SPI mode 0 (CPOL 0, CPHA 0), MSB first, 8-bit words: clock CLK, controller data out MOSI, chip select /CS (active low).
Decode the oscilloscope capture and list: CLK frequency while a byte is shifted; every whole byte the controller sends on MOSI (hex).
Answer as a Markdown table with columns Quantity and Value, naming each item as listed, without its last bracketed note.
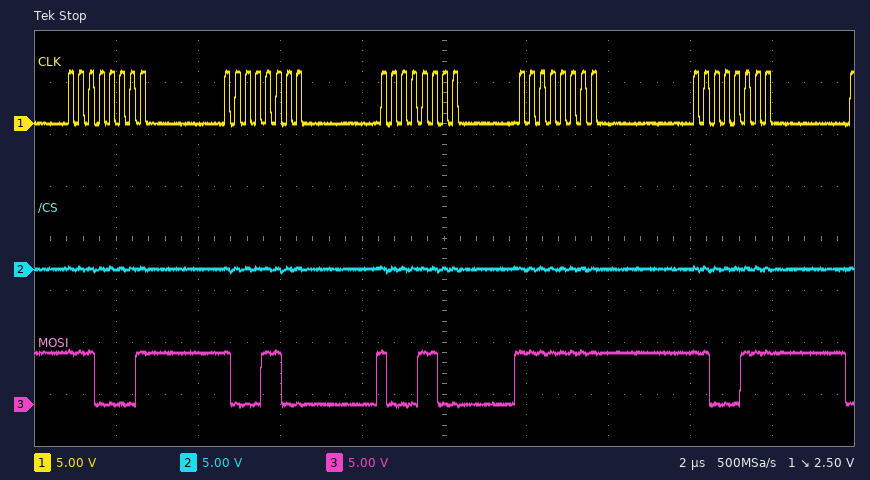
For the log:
| Quantity | Value |
|---|---|
| CLK frequency while a byte is shifted | 4 MHz |
| every whole byte the controller sends on MOSI | E1 8C 8C FF C7 |
